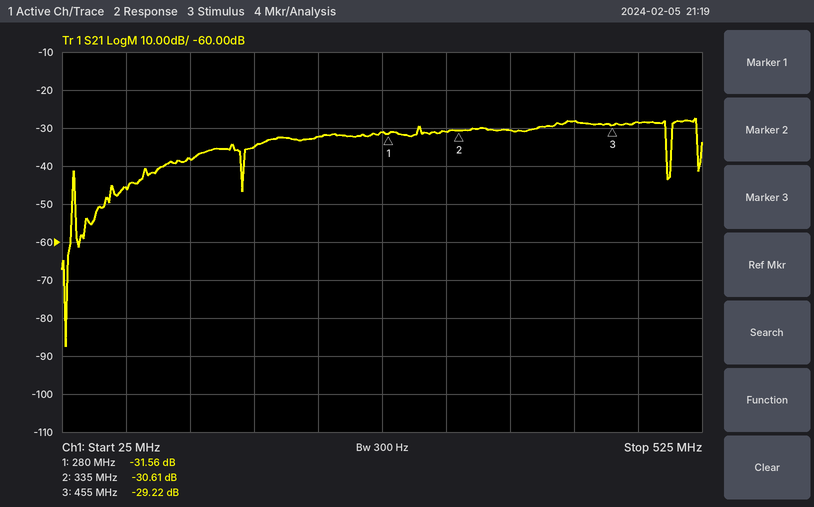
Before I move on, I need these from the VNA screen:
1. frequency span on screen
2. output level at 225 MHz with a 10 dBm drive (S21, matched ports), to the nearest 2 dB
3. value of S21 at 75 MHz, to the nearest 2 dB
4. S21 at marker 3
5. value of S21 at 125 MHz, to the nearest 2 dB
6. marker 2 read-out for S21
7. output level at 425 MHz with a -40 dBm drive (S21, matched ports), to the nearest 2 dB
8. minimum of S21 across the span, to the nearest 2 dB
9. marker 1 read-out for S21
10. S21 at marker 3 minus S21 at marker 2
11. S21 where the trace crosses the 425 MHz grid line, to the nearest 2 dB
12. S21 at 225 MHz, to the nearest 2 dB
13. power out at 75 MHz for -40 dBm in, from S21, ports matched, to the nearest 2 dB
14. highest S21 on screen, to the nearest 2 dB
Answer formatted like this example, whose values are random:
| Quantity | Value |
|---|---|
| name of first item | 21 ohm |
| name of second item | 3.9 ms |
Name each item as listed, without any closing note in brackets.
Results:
| Quantity | Value |
|---|---|
| frequency span on screen | 500 MHz |
| output level at 225 MHz with a 10 dBm drive (S21, matched ports), to the nearest 2 dB | -22 dBm |
| value of S21 at 75 MHz, to the nearest 2 dB | -46 dB |
| S21 at marker 3 | -29.22 dB |
| value of S21 at 125 MHz, to the nearest 2 dB | -38 dB |
| marker 2 read-out for S21 | -30.61 dB |
| output level at 425 MHz with a -40 dBm drive (S21, matched ports), to the nearest 2 dB | -68 dBm |
| minimum of S21 across the span, to the nearest 2 dB | -88 dB |
| marker 1 read-out for S21 | -31.56 dB |
| S21 at marker 3 minus S21 at marker 2 | 1.39 dB |
| S21 where the trace crosses the 425 MHz grid line, to the nearest 2 dB | -28 dB |
| S21 at 225 MHz, to the nearest 2 dB | -32 dB |
| power out at 75 MHz for -40 dBm in, from S21, ports matched, to the nearest 2 dB | -86 dBm |
| highest S21 on screen, to the nearest 2 dB | -28 dB |
